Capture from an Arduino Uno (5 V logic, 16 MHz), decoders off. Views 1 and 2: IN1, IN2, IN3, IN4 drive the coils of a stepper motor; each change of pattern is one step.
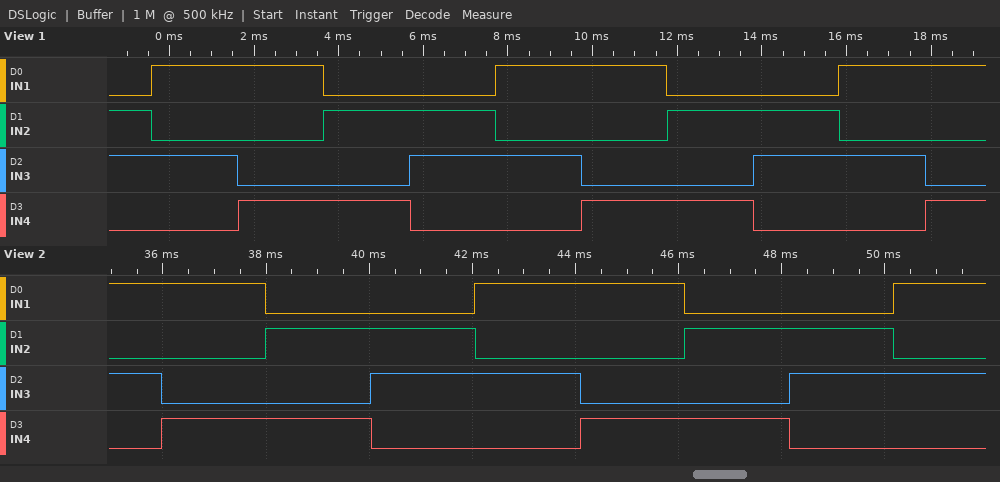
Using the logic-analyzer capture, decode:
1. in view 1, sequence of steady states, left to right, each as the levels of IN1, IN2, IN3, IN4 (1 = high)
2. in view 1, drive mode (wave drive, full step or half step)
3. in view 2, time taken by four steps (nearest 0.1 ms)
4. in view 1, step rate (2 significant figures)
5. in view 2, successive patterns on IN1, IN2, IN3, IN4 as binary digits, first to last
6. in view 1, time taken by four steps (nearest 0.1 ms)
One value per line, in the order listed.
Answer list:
0110 1010 1001 0101 0110 1010 1001 0101 0110 1010 1001
full step
8.1 ms
490 steps/s
1010 1001 0101 0110 1010 1001 0101 0110 1010
8.1 ms
